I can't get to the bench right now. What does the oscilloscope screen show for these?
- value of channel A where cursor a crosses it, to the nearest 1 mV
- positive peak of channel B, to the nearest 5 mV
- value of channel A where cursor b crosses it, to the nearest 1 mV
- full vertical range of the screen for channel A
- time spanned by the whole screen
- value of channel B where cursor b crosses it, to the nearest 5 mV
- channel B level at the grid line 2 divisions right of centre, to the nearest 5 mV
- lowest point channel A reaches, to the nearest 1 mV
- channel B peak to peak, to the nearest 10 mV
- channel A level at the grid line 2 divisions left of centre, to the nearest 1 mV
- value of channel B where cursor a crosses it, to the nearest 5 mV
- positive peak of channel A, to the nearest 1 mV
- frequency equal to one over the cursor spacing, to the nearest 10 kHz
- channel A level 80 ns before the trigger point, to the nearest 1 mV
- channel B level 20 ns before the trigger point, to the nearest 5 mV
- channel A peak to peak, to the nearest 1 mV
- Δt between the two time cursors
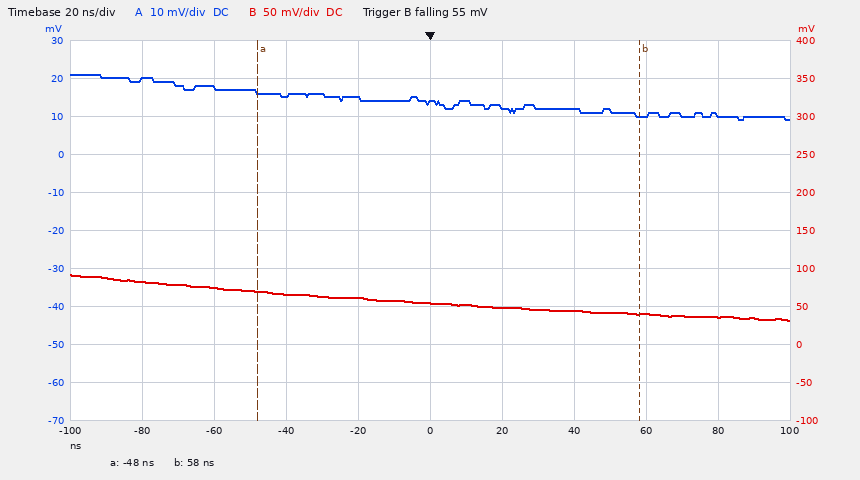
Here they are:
17 mV
90 mV
10 mV
100 mV
200 ns
40 mV
45 mV
9 mV
60 mV
16 mV
70 mV
21 mV
9.43 MHz
20 mV
60 mV
12 mV
106 ns
